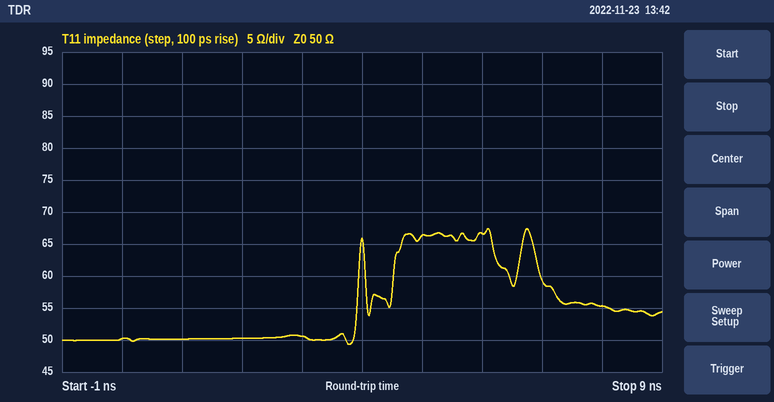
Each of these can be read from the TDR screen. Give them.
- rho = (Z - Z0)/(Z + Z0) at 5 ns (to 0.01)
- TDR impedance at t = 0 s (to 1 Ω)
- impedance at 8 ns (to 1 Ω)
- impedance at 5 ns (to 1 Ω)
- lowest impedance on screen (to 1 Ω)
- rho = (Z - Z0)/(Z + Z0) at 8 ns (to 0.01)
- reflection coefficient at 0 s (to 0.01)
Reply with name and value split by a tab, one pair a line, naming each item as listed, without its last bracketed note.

rho = (Z - Z0)/(Z + Z0) at 5 ns	+0.14
TDR impedance at t = 0 s	50 Ω
impedance at 8 ns	55 Ω
impedance at 5 ns	66 Ω
lowest impedance on screen	49 Ω
rho = (Z - Z0)/(Z + Z0) at 8 ns	+0.05
reflection coefficient at 0 s	0.00
